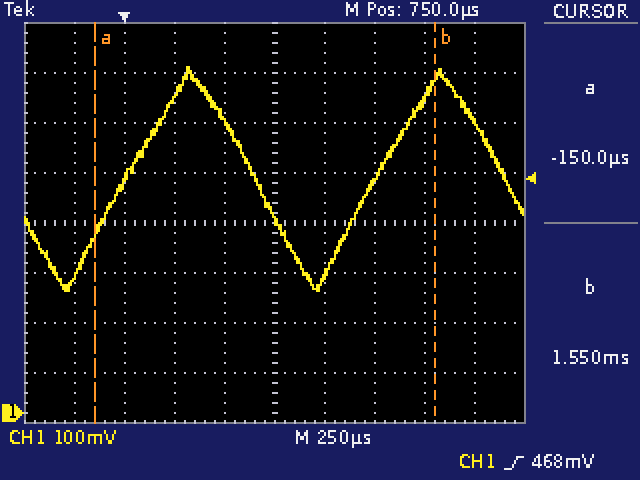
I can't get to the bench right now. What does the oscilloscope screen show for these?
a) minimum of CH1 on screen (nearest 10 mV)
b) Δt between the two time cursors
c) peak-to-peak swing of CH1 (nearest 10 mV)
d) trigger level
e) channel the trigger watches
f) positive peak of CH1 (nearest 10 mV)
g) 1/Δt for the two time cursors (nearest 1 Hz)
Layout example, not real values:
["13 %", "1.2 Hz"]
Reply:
["240 mV", "1.700 ms", "450 mV", "468 mV", "CH1", "690 mV", "588 Hz"]
